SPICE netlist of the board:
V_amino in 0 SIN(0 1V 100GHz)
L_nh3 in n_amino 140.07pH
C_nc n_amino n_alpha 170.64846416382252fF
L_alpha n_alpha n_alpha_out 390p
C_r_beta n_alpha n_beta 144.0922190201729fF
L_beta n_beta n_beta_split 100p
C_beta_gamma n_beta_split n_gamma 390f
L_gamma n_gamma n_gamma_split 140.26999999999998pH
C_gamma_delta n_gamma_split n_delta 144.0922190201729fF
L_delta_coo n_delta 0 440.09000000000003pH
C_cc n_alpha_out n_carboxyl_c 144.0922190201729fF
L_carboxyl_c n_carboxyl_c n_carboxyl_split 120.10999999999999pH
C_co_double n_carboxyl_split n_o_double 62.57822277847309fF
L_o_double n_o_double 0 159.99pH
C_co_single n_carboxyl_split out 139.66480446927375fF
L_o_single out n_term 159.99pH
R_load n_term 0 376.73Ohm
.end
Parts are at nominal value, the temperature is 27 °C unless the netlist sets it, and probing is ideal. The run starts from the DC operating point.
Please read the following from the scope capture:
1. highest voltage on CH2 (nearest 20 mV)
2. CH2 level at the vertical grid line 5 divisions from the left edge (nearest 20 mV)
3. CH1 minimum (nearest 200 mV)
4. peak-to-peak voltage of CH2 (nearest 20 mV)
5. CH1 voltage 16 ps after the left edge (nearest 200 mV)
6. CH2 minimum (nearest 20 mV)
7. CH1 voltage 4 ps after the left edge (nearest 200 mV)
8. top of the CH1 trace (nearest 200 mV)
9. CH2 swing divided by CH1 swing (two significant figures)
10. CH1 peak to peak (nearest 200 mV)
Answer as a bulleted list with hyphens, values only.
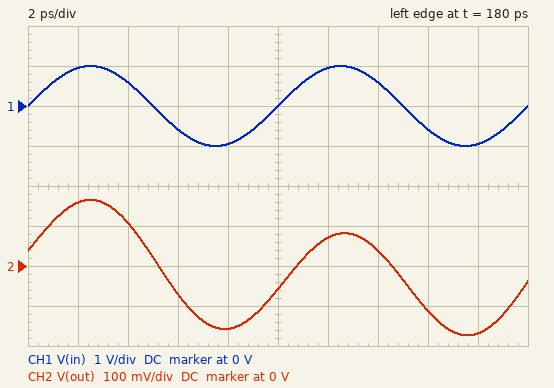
- 160 mV
- -60 mV
- -1.0 V
- 340 mV
- -600 mV
- -180 mV
- 600 mV
- 1.0 V
- 0.17
- 2.0 V
